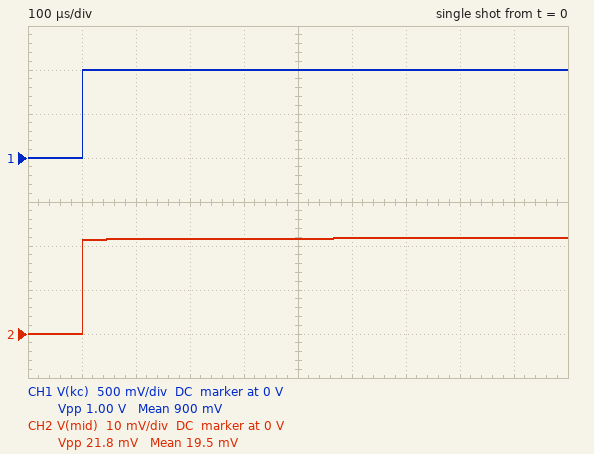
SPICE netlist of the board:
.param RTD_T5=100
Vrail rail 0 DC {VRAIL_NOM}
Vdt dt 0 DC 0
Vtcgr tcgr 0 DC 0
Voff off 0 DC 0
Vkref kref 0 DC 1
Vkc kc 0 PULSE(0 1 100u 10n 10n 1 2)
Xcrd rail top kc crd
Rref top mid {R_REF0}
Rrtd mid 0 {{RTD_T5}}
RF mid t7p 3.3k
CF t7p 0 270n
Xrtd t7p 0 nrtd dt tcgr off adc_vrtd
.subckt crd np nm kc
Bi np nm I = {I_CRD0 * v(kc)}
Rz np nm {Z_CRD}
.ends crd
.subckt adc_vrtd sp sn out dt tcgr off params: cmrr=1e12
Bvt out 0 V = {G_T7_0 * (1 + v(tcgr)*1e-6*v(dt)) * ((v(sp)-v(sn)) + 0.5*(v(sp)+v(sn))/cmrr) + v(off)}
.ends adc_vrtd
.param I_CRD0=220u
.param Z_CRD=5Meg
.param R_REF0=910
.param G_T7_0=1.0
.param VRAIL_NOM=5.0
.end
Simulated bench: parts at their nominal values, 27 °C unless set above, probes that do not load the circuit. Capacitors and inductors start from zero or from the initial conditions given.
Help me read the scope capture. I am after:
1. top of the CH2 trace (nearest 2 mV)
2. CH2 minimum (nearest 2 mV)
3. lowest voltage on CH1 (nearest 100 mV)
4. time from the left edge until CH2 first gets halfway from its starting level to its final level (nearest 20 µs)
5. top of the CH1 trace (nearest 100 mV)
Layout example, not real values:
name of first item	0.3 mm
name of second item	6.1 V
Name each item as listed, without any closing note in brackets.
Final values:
top of the CH2 trace	22 mV
CH2 minimum	0 V
lowest voltage on CH1	0 V
time from the left edge until CH2 first gets halfway from its starting level to its final level	100 µs
top of the CH1 trace	1.0 V
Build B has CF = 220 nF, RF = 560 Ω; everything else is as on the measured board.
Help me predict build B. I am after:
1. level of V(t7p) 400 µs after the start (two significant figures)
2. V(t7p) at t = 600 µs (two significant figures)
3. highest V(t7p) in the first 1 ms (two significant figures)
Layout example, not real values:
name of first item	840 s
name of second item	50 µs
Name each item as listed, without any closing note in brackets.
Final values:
level of V(t7p) 400 µs after the start	19 mV
V(t7p) at t = 600 µs	21 mV
highest V(t7p) in the first 1 ms	22 mV
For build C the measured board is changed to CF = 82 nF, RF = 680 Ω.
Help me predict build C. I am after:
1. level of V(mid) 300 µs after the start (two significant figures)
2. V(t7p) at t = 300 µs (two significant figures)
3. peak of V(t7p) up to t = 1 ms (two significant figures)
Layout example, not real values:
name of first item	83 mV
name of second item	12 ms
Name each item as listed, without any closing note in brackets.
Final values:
level of V(mid) 300 µs after the start	22 mV
V(t7p) at t = 300 µs	21 mV
peak of V(t7p) up to t = 1 ms	22 mV
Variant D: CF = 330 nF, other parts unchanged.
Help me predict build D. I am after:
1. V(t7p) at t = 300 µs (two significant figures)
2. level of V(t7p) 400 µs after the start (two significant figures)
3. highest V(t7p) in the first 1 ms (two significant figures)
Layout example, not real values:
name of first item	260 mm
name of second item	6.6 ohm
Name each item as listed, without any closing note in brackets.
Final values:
V(t7p) at t = 300 µs	3.6 mV
level of V(t7p) 400 µs after the start	5.2 mV
highest V(t7p) in the first 1 ms	12 mV
